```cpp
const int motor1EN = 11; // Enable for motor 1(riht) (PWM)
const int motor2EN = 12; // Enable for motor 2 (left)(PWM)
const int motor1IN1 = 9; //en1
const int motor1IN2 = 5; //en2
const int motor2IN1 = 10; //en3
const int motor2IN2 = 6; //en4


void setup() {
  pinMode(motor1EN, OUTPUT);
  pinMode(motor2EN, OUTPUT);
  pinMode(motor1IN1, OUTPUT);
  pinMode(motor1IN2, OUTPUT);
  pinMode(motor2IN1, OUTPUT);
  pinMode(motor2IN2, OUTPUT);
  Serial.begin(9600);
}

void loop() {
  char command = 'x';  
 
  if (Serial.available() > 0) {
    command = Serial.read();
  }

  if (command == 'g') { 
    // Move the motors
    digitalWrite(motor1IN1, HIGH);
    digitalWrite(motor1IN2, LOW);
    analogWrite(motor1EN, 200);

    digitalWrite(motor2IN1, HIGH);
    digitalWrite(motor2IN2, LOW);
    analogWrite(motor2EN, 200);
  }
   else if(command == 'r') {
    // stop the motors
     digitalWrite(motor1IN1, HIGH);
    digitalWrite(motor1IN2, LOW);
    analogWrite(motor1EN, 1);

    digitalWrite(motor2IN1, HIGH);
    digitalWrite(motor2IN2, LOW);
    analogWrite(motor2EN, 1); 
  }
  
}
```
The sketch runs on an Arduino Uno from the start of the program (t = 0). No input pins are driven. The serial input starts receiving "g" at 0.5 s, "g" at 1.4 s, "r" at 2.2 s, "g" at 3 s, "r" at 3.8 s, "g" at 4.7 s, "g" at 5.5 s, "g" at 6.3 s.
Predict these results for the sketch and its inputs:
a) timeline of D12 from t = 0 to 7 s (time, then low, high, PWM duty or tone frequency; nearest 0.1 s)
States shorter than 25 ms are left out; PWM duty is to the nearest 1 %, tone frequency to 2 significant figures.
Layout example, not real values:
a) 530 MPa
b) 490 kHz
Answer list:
a) 0 s low; 0.5 s high; 2.2 s low; 3 s high; 3.8 s low; 4.7 s high
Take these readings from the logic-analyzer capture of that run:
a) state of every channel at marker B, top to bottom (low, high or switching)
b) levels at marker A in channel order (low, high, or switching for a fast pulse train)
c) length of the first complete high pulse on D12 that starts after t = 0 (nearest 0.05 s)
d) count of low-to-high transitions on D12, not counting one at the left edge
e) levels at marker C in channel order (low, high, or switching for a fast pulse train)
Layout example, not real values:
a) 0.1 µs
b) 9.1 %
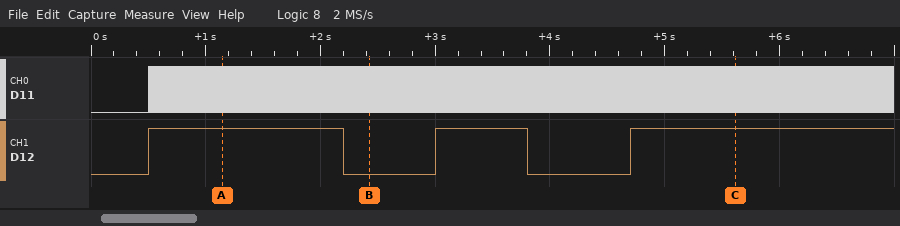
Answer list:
a) D11 switching, D12 low
b) D11 switching, D12 high
c) 1.70 s
d) 3
e) D11 switching, D12 high
